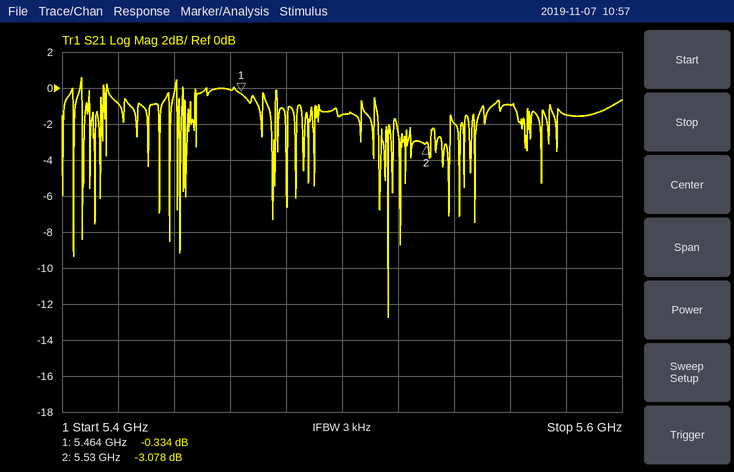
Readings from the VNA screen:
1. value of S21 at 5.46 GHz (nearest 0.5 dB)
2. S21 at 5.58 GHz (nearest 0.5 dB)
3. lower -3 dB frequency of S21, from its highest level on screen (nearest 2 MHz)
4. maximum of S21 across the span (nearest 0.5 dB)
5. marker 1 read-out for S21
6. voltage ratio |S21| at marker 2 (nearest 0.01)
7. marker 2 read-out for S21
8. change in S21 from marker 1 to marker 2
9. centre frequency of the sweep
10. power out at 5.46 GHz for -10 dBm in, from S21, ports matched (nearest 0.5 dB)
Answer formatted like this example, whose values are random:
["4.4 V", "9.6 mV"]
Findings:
["0.0 dB", "-1.5 dB", "5.404 GHz", "0.5 dB", "-0.334 dB", "0.70", "-3.078 dB", "-2.744 dB", "5.5 GHz", "-10.0 dBm"]
